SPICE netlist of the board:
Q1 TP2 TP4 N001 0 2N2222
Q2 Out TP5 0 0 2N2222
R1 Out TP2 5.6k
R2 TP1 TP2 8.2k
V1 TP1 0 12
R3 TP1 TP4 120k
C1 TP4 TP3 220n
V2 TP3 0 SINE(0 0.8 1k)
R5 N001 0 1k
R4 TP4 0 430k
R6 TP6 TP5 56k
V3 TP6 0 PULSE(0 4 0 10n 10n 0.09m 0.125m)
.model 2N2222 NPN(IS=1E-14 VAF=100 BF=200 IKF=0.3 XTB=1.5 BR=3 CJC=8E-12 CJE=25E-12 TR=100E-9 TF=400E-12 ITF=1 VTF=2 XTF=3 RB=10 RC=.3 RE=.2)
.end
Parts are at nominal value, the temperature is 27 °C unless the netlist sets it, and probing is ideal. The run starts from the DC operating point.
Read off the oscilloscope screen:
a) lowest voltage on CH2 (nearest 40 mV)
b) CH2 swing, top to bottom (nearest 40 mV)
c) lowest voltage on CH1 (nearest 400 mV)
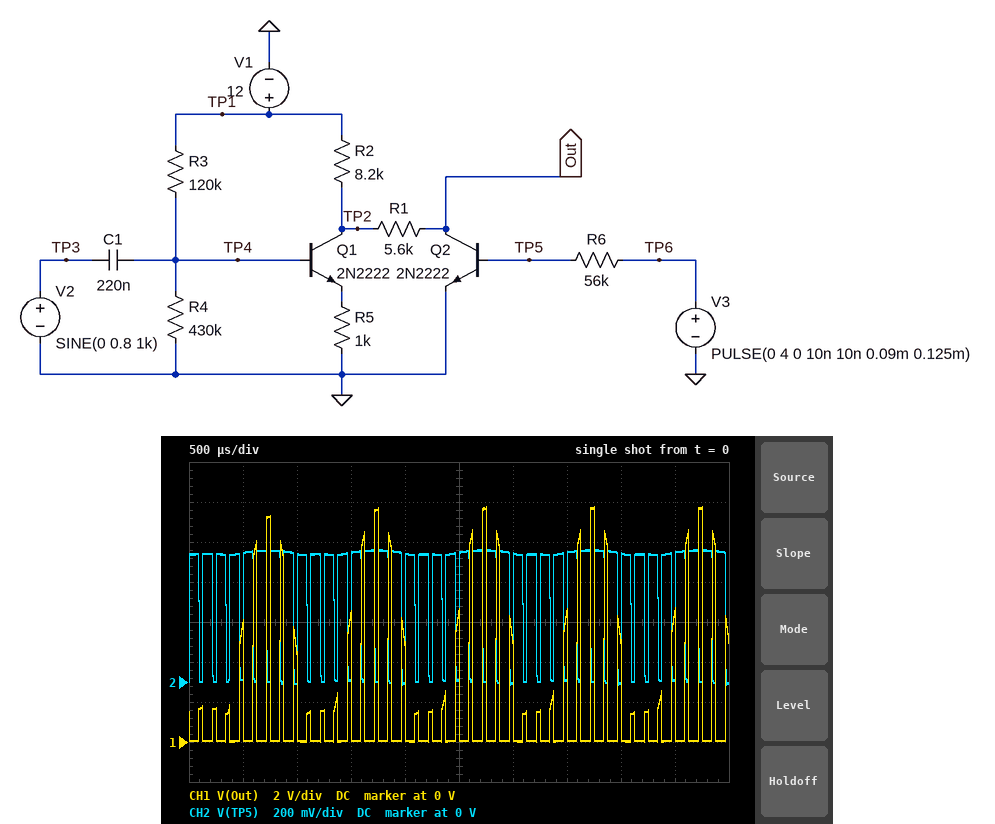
0 V
680 mV
0 V
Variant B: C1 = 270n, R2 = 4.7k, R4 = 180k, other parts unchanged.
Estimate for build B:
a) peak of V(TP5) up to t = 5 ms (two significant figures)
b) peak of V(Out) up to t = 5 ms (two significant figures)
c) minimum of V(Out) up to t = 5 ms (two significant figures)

660 mV
9.2 V
29 mV
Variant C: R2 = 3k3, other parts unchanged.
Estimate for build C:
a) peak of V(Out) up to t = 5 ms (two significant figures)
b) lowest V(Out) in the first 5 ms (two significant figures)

8.1 V
34 mV
